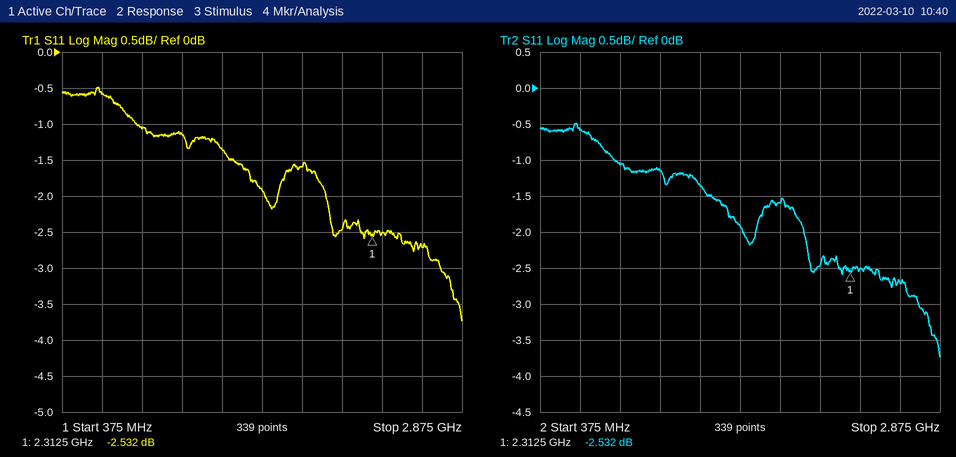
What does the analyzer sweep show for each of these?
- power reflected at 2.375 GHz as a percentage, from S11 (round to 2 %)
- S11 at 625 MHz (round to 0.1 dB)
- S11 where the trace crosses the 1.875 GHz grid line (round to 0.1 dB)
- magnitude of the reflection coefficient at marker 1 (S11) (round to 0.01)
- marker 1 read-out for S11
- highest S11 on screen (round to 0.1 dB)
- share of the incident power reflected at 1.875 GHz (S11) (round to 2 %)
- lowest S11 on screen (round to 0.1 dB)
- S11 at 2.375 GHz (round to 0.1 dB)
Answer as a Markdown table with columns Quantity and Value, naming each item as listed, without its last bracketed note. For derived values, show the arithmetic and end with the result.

| Quantity | Value |
|---|---|
| power reflected at 2.375 GHz as a percentage, from S11 | 10^(-2.5/10) ≈ 56 % |
| S11 at 625 MHz | -0.6 dB |
| S11 where the trace crosses the 1.875 GHz grid line | -1.6 dB |
| magnitude of the reflection coefficient at marker 1 (S11) | 10^(-2.532/20) ≈ 0.75 |
| marker 1 read-out for S11 | -2.532 dB |
| highest S11 on screen | -0.5 dB |
| share of the incident power reflected at 1.875 GHz (S11) | 10^(-1.6/10) ≈ 69.2 %, so 70 % to the nearest 2 % |
| lowest S11 on screen | -3.7 dB |
| S11 at 2.375 GHz | -2.5 dB |
